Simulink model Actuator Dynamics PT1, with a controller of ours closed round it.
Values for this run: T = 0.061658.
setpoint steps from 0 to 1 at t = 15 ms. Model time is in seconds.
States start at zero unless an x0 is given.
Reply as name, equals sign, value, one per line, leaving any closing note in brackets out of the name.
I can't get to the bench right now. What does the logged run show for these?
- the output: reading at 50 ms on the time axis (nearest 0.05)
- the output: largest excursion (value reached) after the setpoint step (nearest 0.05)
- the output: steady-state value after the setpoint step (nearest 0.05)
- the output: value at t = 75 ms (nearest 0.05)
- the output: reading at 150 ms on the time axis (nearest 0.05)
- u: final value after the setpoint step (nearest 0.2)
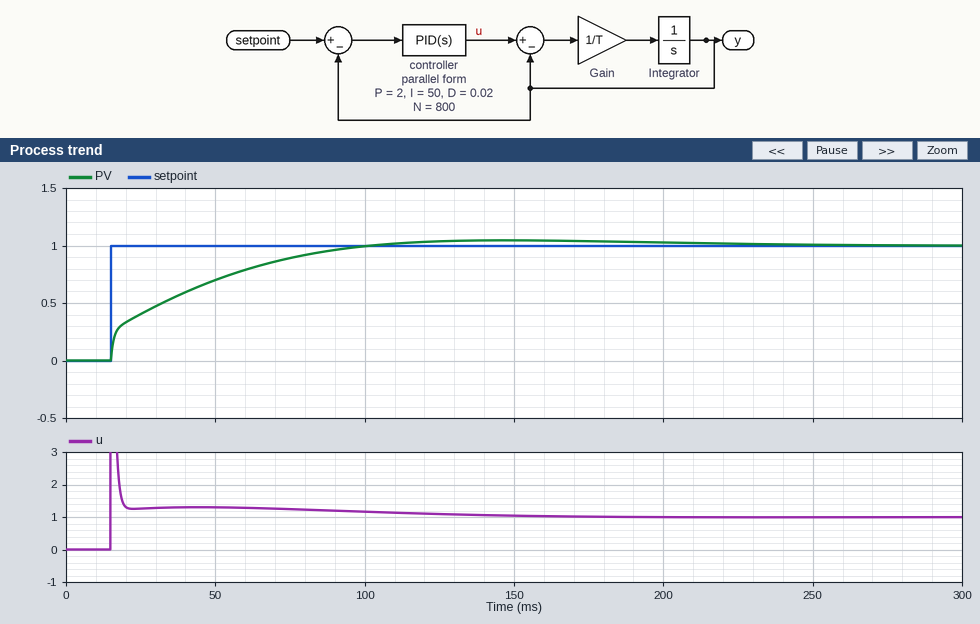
the output: reading at 50 ms on the time axis = 0.70
the output: largest excursion (value reached) after the setpoint step = 1.05
the output: steady-state value after the setpoint step = 1.00
the output: value at t = 75 ms = 0.90
the output: reading at 150 ms on the time axis = 1.05
u: final value after the setpoint step = 1.0
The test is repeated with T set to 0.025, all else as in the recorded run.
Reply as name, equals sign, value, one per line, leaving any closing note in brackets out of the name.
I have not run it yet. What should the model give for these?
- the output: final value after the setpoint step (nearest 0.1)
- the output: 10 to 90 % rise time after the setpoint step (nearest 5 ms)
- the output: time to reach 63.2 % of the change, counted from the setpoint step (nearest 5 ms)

the output: final value after the setpoint step = 1.0
the output: 10 to 90 % rise time after the setpoint step = 60 ms
the output: time to reach 63.2 % of the change, counted from the setpoint step = 15 ms
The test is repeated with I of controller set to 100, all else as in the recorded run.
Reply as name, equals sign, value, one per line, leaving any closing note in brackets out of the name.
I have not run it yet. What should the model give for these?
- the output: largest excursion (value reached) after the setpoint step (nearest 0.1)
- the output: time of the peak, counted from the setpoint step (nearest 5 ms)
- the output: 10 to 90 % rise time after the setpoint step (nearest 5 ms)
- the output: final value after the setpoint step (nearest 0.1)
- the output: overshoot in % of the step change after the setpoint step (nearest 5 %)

the output: largest excursion (value reached) after the setpoint step = 1.1
the output: time of the peak, counted from the setpoint step = 85 ms
the output: 10 to 90 % rise time after the setpoint step = 40 ms
the output: final value after the setpoint step = 1.0
the output: overshoot in % of the step change after the setpoint step = 15 %
